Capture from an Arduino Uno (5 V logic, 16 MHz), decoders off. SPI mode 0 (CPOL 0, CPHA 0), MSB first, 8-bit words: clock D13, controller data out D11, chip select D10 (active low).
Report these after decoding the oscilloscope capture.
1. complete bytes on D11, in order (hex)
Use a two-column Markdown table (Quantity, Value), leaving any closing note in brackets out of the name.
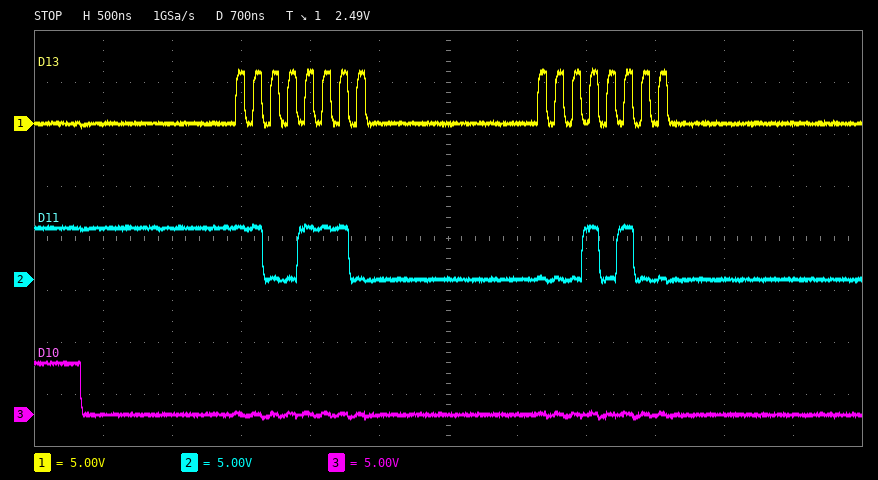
| Quantity | Value |
|---|---|
| complete bytes on D11, in order | 0xCE 0x14 |
